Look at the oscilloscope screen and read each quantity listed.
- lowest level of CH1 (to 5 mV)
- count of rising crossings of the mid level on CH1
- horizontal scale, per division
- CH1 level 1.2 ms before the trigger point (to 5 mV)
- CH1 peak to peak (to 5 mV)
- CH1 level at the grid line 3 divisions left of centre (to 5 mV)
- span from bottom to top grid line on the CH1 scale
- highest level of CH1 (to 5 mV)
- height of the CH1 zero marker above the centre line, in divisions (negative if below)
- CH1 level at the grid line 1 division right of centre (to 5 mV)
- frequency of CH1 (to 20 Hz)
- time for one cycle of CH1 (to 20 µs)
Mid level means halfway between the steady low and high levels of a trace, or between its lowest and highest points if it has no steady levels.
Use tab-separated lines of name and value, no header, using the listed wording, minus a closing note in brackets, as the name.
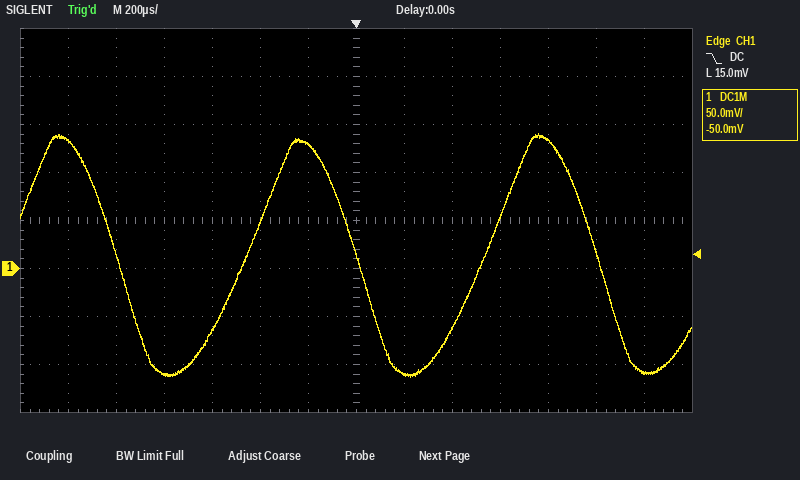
lowest level of CH1	-115 mV
count of rising crossings of the mid level on CH1	2
horizontal scale, per division	200 µs
CH1 level 1.2 ms before the trigger point	135 mV
CH1 peak to peak	255 mV
CH1 level at the grid line 3 divisions left of centre	-65 mV
span from bottom to top grid line on the CH1 scale	400 mV
highest level of CH1	140 mV
height of the CH1 zero marker above the centre line, in divisions	-1.0 div
CH1 level at the grid line 1 division right of centre	-110 mV
frequency of CH1	1.00 kHz
time for one cycle of CH1	1.00 ms
